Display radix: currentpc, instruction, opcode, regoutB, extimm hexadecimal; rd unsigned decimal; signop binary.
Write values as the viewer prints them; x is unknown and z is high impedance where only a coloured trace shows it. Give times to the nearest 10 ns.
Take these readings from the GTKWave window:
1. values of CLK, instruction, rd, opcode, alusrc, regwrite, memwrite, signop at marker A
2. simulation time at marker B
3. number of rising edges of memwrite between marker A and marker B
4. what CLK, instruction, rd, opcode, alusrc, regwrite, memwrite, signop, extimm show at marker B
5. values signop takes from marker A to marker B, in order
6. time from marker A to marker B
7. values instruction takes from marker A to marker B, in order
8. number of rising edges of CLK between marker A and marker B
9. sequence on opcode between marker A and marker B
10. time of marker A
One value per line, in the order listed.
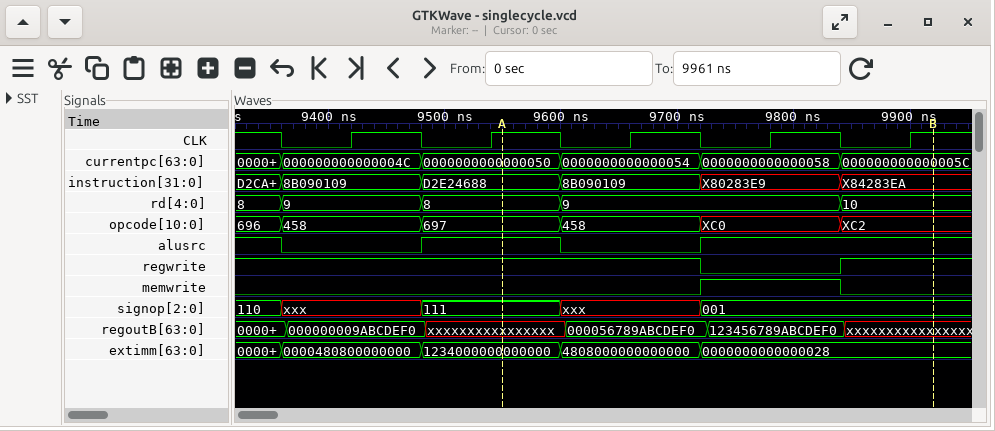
CLK=1, instruction=D2E24688, rd=8, opcode=697, alusrc=1, regwrite=1, memwrite=0, signop=111
9920 ns
1
CLK=1, instruction=X84283EA, rd=10, opcode=XC2, alusrc=1, regwrite=1, memwrite=0, signop=001, extimm=0000000000000028
111, xxx, 001
370 ns
D2E24688, 8B090109, X80283E9, X84283EA
3
697, 458, XC0, XC2
9550 ns
